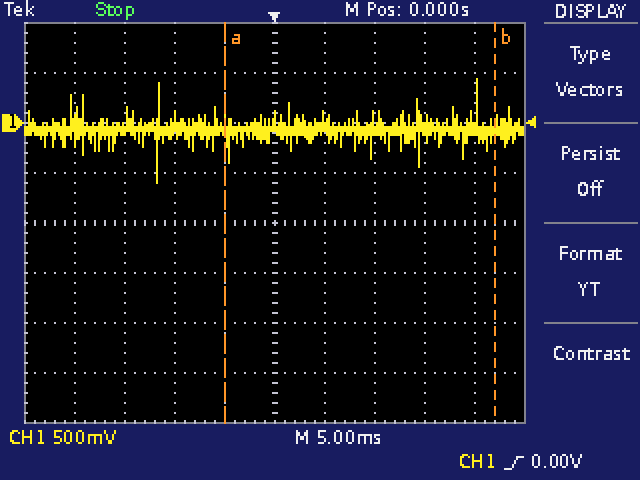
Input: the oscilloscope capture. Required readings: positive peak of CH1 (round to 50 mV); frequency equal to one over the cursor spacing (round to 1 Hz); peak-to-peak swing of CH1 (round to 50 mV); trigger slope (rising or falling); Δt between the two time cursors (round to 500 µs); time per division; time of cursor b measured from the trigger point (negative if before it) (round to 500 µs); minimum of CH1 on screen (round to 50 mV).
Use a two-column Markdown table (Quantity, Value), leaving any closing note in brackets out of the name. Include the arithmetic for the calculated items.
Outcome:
| Quantity | Value |
|---|---|
| positive peak of CH1 | 450 mV |
| frequency equal to one over the cursor spacing | 1 / 27.0 ms ≈ 37 Hz |
| peak-to-peak swing of CH1 | 450 mV − (-600 mV) = 1.05 V |
| trigger slope | rising |
| Δt between the two time cursors | 27.0 ms |
| time per division | 5 ms |
| time of cursor b measured from the trigger point (negative if before it) | +22.0 ms |
| minimum of CH1 on screen | -600 mV |
